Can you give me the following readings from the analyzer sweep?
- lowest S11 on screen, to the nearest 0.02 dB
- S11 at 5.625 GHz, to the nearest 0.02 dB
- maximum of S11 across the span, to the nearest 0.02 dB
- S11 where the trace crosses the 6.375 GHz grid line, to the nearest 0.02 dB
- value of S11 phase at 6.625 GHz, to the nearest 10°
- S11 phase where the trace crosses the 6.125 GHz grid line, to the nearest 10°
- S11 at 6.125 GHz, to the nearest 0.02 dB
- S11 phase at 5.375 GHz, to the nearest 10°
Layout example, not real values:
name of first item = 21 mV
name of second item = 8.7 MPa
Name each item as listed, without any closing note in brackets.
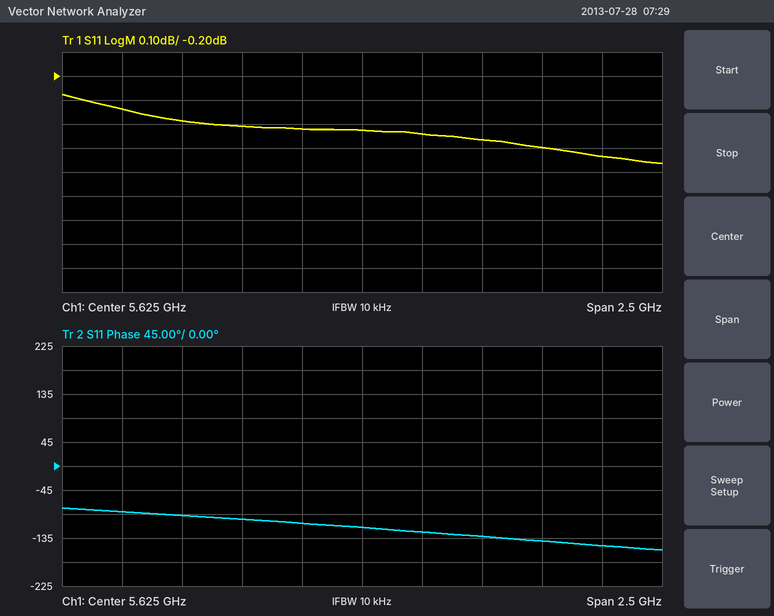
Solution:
lowest S11 on screen, to the nearest 0.02 dB = -0.56 dB
S11 at 5.625 GHz, to the nearest 0.02 dB = -0.42 dB
maximum of S11 across the span, to the nearest 0.02 dB = -0.28 dB
S11 where the trace crosses the 6.375 GHz grid line, to the nearest 0.02 dB = -0.50 dB
value of S11 phase at 6.625 GHz, to the nearest 10° = -150°
S11 phase where the trace crosses the 6.125 GHz grid line, to the nearest 10° = -130°
S11 at 6.125 GHz, to the nearest 0.02 dB = -0.46 dB
S11 phase at 5.375 GHz, to the nearest 10° = -110°
